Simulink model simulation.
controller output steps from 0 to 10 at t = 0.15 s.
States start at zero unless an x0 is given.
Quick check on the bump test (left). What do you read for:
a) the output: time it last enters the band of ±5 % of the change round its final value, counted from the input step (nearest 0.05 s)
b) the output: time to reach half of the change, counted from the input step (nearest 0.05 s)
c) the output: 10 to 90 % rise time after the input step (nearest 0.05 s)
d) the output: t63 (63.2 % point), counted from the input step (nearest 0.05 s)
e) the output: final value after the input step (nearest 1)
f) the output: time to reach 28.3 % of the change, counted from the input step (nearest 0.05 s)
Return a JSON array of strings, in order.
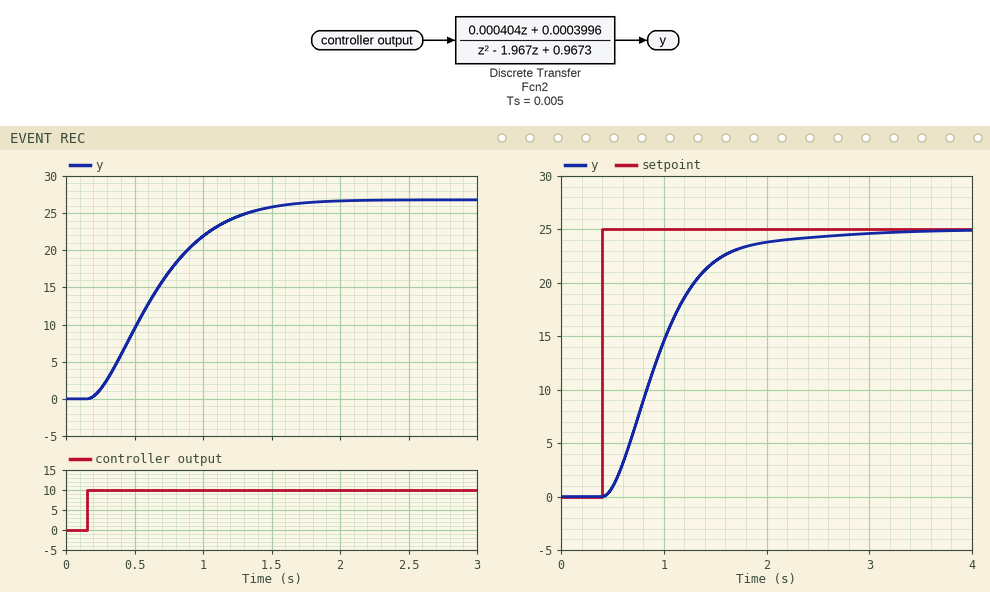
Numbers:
["1.25 s", "0.45 s", "0.90 s", "0.60 s", "27", "0.30 s"]
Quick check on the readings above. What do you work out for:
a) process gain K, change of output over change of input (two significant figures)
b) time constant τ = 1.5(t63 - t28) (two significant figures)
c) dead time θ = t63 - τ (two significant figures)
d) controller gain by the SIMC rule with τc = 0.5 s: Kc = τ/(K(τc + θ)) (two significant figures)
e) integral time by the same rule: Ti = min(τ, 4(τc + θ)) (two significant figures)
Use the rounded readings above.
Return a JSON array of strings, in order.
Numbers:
["2.7", "0.45 s", "0.15 s", "0.26", "0.45 s"]
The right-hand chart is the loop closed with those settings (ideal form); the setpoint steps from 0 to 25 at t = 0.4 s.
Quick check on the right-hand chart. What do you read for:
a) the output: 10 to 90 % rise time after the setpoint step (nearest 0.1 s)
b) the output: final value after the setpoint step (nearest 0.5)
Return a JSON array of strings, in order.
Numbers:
["1.0 s", "25.0"]
